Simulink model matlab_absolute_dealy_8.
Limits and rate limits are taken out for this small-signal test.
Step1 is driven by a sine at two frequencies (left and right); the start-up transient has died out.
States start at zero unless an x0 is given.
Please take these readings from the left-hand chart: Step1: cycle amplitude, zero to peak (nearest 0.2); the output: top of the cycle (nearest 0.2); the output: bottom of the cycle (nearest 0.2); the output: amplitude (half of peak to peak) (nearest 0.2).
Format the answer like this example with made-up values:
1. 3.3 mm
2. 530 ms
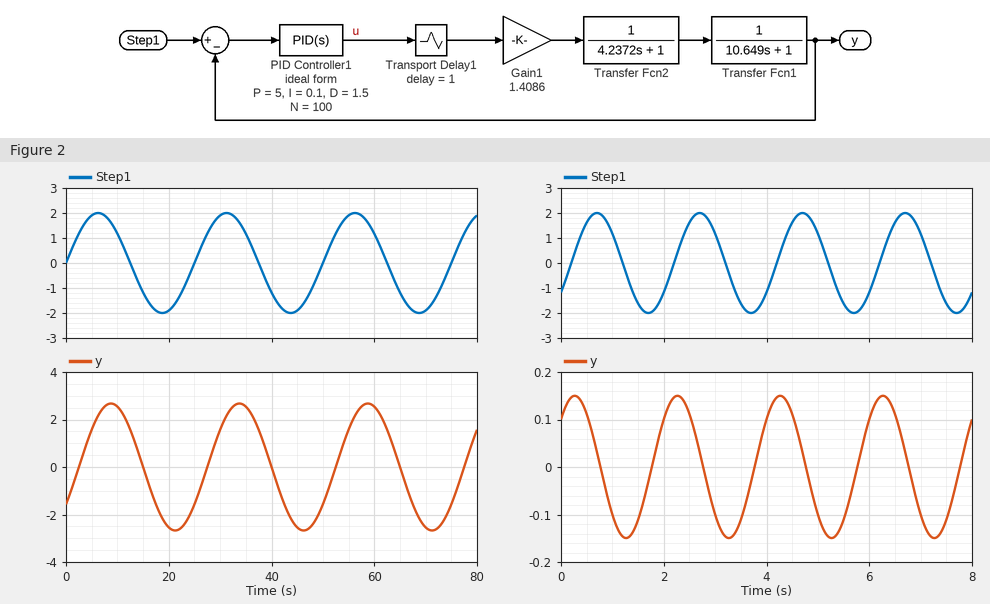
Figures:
1. 2.0
2. 2.6
3. -2.6
4. 2.6
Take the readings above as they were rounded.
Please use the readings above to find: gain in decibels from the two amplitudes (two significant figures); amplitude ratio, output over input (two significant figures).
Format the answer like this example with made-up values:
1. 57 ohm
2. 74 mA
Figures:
1. 2.3 dB
2. 1.3
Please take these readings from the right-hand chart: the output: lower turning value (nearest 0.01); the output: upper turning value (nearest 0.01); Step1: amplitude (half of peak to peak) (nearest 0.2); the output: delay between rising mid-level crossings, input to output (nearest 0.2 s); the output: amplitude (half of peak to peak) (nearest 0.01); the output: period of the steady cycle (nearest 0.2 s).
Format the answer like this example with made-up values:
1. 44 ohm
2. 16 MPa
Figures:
1. -0.15
2. 0.15
3. 2.0
4. 1.6 s
5. 0.15
6. 2.0 s
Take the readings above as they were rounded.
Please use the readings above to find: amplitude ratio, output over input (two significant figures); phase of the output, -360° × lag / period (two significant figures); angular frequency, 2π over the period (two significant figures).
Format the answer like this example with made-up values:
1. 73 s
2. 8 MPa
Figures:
1. 0.075
2. -290°
3. 3.1 rad/s
